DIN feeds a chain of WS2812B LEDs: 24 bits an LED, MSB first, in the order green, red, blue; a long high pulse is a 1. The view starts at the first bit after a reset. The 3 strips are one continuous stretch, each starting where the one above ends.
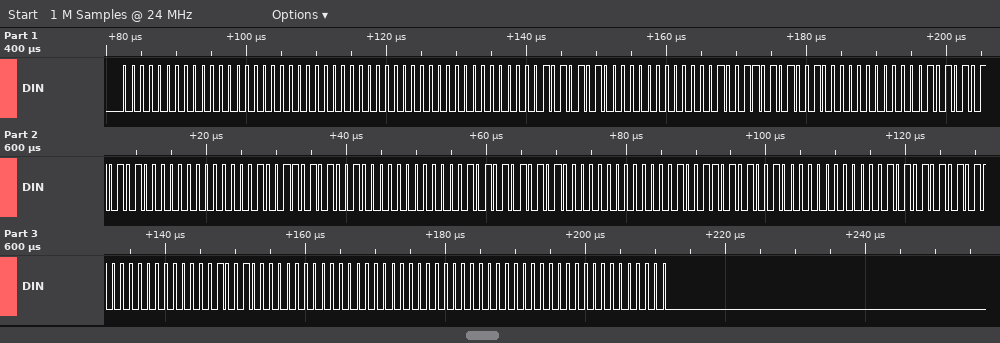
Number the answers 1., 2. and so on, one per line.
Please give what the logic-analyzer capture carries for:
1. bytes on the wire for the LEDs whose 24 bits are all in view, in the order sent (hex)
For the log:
1. 00 00 00 00 00 00 AA 00 09 A9 00 0A AA 00 09 A9 00 0A AA 00 09 A9 00 0A AA 00 09 00 00 00 00 00 00
